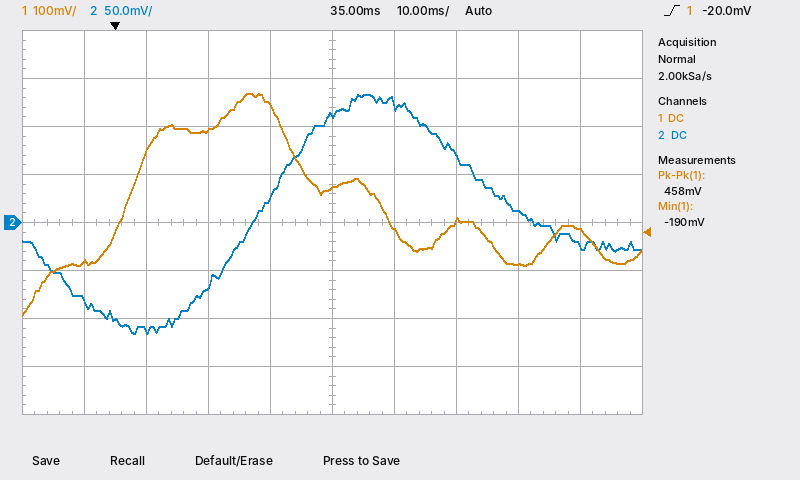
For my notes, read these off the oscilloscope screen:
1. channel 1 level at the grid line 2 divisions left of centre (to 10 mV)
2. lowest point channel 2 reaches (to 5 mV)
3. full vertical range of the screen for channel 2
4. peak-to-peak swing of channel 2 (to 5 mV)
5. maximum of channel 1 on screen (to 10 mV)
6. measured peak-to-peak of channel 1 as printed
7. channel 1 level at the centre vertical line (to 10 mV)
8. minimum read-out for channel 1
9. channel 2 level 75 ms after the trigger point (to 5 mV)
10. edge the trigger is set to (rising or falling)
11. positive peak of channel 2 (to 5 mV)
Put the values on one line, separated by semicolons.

190 mV; -115 mV; 400 mV; 250 mV; 270 mV; 458 mV; 70 mV; -190 mV; -25 mV; rising; 135 mV
